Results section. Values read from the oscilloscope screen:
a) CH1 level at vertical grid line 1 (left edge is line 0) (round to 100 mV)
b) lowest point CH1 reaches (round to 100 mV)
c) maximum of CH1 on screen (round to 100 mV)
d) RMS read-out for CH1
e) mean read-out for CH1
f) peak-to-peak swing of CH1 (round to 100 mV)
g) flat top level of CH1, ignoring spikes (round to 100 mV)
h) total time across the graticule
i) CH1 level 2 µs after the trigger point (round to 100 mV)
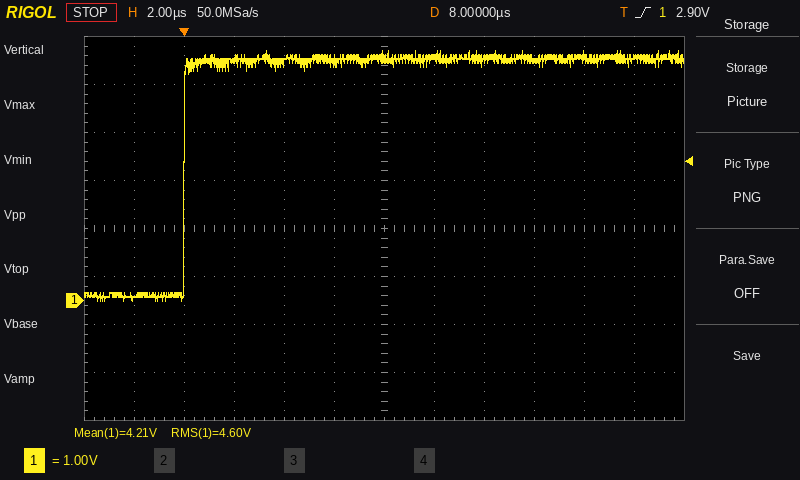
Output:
100 mV
0.0 V
5.2 V
4.60 V
4.21 V
5.2 V
5.0 V
24 µs
5.0 V
